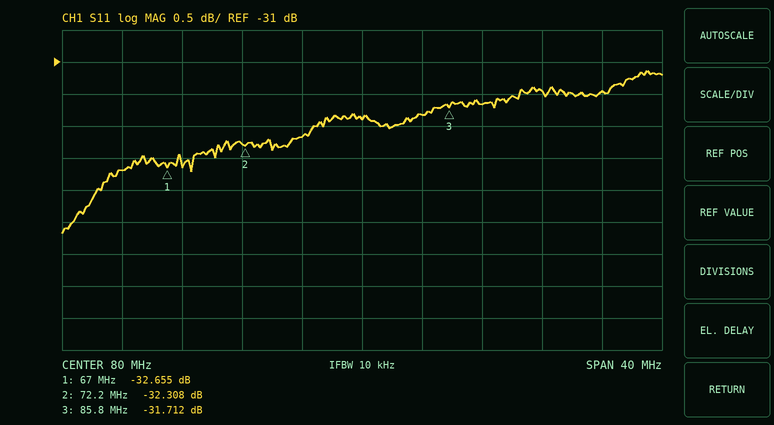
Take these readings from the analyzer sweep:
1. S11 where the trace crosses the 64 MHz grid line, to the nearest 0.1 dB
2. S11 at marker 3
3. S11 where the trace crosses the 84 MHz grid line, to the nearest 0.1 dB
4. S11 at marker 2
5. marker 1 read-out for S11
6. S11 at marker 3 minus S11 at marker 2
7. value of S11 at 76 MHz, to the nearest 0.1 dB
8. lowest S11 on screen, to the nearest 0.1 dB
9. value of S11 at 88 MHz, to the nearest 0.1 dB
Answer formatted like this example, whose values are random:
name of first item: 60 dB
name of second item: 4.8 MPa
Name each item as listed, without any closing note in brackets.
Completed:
S11 where the trace crosses the 64 MHz grid line, to the nearest 0.1 dB: -32.7 dB
S11 at marker 3: -31.712 dB
S11 where the trace crosses the 84 MHz grid line, to the nearest 0.1 dB: -31.8 dB
S11 at marker 2: -32.308 dB
marker 1 read-out for S11: -32.655 dB
S11 at marker 3 minus S11 at marker 2: 0.596 dB
value of S11 at 76 MHz, to the nearest 0.1 dB: -32.2 dB
lowest S11 on screen, to the nearest 0.1 dB: -33.7 dB
value of S11 at 88 MHz, to the nearest 0.1 dB: -31.7 dB
